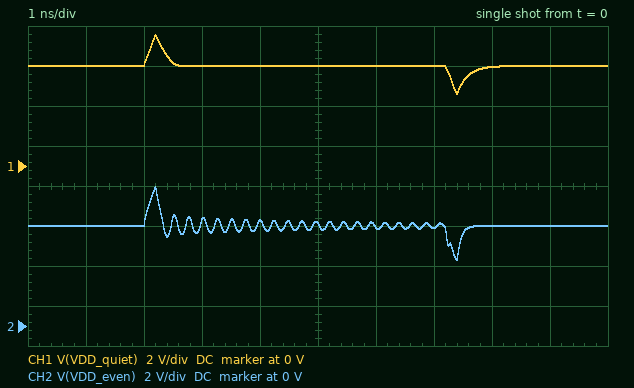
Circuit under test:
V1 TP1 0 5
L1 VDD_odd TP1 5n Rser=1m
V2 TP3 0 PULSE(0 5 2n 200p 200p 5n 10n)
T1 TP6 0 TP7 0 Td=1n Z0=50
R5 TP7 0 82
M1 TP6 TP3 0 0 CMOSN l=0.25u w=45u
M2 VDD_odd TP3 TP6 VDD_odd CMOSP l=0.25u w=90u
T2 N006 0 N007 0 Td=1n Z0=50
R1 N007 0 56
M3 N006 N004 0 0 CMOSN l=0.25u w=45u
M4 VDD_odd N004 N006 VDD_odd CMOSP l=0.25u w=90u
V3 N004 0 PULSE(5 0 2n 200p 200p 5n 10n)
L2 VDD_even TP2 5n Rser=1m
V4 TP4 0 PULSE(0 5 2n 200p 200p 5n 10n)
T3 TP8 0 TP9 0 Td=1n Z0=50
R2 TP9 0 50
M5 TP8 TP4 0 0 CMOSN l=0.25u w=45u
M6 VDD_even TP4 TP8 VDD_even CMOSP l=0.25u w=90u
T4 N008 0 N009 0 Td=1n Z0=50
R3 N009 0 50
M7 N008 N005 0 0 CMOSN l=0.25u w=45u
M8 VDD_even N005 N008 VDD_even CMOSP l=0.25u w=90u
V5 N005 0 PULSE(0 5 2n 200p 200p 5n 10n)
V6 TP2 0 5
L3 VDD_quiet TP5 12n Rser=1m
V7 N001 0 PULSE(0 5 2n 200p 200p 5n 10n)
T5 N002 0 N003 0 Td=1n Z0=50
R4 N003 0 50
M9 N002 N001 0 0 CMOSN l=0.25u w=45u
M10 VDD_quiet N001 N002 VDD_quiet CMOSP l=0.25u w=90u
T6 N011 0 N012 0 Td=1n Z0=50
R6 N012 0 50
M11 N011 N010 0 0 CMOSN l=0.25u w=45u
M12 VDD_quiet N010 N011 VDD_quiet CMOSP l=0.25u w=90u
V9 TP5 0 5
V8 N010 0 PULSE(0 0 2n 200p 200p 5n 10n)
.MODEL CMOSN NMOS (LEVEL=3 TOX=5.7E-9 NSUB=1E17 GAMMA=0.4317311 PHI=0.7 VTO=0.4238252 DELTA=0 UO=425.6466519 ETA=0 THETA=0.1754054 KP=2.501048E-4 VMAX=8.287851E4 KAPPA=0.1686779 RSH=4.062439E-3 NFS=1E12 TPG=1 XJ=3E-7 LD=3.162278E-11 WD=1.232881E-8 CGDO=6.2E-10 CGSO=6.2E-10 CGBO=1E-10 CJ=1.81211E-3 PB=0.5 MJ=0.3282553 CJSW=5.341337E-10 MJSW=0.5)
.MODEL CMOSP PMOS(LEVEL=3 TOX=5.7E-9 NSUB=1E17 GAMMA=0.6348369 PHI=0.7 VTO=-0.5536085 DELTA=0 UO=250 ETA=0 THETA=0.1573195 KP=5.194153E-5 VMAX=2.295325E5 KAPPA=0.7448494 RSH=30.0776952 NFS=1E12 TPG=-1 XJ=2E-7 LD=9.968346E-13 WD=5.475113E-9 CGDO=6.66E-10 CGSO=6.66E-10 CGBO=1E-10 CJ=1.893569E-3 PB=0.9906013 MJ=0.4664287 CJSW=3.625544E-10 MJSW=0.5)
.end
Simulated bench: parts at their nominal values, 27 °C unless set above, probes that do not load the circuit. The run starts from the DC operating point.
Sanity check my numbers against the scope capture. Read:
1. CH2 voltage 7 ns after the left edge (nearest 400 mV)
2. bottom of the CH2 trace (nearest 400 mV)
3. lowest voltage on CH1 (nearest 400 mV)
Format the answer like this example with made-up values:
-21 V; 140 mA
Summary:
4.8 V; 3.2 V; 3.6 V
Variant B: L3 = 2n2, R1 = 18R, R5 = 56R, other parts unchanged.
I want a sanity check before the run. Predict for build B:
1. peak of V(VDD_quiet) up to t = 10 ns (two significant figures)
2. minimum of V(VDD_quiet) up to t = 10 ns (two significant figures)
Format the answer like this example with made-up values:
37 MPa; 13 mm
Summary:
5.5 V; 4.5 V
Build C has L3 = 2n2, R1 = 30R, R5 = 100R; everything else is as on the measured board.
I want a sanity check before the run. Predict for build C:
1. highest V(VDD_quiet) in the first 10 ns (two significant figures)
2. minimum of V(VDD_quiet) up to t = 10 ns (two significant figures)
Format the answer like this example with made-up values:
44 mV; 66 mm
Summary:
5.5 V; 4.5 V
